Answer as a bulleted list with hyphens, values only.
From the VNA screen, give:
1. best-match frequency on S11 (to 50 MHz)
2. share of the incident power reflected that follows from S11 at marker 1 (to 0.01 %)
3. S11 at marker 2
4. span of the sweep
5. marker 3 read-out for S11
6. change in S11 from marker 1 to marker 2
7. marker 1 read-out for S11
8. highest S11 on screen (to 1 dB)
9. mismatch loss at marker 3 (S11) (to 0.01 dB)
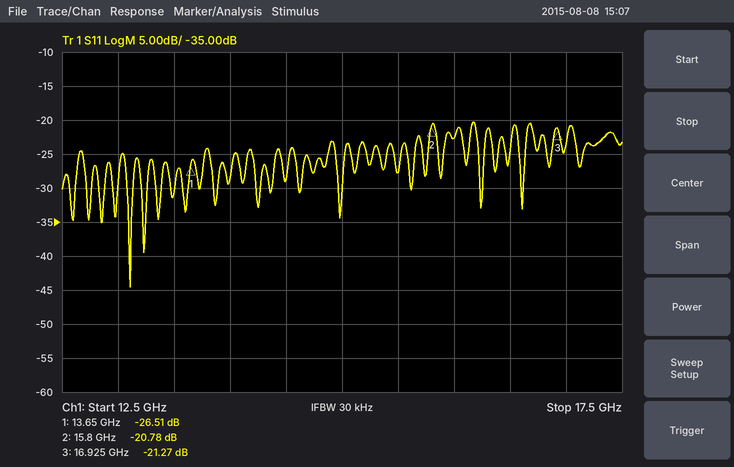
- 13.10 GHz
- 0.22 %
- -20.78 dB
- 5 GHz
- -21.27 dB
- 5.73 dB
- -26.51 dB
- -20 dB
- 0.03 dB
